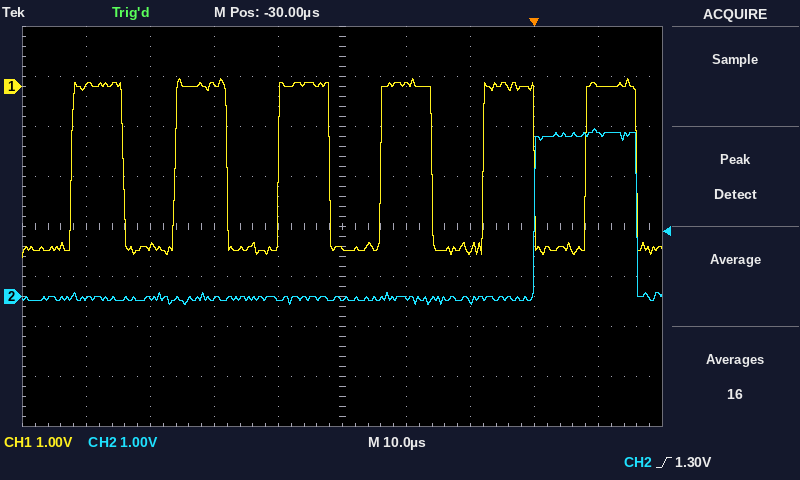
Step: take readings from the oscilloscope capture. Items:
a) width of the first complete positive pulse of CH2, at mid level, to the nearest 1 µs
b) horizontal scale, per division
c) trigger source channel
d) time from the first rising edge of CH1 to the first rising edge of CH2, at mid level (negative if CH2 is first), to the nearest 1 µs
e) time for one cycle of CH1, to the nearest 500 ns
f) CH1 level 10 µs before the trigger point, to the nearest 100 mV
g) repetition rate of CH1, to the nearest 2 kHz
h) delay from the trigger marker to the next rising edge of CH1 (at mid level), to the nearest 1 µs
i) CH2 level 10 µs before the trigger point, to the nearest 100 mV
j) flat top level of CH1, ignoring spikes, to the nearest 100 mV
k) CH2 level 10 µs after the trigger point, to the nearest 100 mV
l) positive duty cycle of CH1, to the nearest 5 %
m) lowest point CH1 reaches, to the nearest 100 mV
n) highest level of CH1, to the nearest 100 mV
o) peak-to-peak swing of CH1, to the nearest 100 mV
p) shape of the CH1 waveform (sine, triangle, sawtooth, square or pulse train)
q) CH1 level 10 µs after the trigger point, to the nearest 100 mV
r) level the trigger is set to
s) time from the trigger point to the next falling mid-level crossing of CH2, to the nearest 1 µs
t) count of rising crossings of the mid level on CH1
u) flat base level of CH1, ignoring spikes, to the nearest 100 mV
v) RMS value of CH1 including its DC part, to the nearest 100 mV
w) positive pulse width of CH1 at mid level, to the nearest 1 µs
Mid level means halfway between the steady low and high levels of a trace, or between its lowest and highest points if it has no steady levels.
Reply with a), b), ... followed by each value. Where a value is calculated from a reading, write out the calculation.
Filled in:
a) 16 µs
b) 10 µs
c) CH2
d) +72 µs
e) 16.0 µs
f) -3.3 V
g) 1 / 16.0 µs ≈ 62 kHz
h) 8 µs
i) -100 mV
j) 0.0 V
k) 3.3 V
l) 8 µs / 16.0 µs ≈ 50 %
m) -3.4 V
n) 200 mV
o) 200 mV − (-3.4 V) = 3.6 V
p) square
q) 0.0 V
r) 1.30 V
s) 16 µs
t) 6
u) -3.3 V
v) √(0.5 × (0.0 V)² + 0.5 × (-3.3 V)²) ≈ 2.3 V
w) 8 µs
